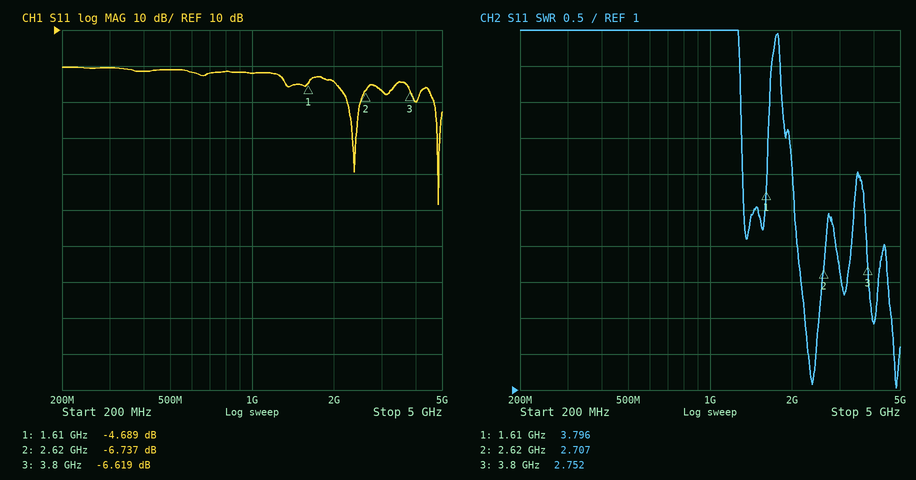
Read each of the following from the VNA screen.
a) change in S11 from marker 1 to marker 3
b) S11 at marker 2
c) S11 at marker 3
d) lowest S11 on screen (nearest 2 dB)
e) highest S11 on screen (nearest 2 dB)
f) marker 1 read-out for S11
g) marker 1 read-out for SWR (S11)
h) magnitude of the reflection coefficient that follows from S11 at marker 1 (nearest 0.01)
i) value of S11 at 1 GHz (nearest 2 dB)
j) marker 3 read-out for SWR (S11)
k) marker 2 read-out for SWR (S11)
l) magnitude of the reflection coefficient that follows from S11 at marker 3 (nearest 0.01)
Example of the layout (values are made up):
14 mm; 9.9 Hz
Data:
-1.930 dB; -6.737 dB; -6.619 dB; -38 dB; 0 dB; -4.689 dB; 3.796; 0.58; -2 dB; 2.752; 2.707; 0.47
